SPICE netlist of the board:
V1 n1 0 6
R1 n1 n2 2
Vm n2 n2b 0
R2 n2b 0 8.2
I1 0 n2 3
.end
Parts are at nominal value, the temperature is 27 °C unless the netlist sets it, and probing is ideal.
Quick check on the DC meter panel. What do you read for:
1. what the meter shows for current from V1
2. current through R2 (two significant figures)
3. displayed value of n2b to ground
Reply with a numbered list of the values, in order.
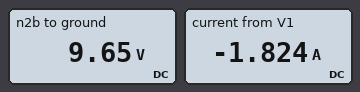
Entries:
1. -1.824 A
2. 1.2 A
3. 9.65 V
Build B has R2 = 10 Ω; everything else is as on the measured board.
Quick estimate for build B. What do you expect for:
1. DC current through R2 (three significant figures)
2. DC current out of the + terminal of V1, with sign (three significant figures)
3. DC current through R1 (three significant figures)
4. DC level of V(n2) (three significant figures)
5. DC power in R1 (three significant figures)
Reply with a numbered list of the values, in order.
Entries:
1. 1.00 A
2. -2.00 A
3. 2.00 A
4. 10.0 V
5. 8.00 W
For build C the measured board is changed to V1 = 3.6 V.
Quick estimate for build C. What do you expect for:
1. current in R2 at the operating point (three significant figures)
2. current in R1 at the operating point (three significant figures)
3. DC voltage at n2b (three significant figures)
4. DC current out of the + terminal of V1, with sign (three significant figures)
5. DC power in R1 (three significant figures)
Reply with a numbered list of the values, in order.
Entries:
1. 941 mA
2. 2.06 A
3. 7.72 V
4. -2.06 A
5. 8.48 W
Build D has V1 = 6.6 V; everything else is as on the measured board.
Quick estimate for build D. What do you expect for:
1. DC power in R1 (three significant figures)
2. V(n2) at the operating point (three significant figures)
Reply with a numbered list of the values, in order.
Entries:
1. 6.23 W
2. 10.1 V
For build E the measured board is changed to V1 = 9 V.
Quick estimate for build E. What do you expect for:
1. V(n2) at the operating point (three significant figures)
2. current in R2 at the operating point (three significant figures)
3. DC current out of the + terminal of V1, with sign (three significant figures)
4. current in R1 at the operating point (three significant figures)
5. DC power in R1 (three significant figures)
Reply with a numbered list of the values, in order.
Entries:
1. 12.1 V
2. 1.47 A
3. -1.53 A
4. 1.53 A
5. 4.68 W
